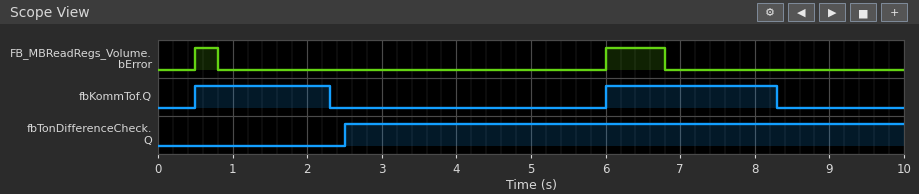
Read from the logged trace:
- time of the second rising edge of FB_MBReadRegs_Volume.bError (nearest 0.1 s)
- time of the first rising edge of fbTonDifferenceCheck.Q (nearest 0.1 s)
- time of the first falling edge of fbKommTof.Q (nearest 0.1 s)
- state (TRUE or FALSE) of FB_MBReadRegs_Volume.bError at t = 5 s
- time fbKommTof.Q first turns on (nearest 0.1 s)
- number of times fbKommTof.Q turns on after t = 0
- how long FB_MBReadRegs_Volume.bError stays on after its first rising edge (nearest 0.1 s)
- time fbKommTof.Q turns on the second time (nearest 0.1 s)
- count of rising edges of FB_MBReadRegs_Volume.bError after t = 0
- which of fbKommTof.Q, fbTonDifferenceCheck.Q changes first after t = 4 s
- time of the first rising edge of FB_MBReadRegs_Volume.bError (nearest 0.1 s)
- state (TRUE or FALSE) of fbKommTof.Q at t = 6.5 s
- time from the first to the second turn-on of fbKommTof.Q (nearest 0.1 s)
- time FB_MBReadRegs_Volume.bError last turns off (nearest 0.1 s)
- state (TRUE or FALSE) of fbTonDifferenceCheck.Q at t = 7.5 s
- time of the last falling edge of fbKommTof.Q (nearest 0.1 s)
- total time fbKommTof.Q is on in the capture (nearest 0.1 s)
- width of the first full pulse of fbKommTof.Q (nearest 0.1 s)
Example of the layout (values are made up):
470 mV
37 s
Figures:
6.0 s
2.5 s
2.3 s
FALSE
0.5 s
2
0.3 s
6.0 s
2
fbKommTof.Q
0.5 s
TRUE
5.5 s
6.8 s
TRUE
8.3 s
4.1 s
1.8 s
